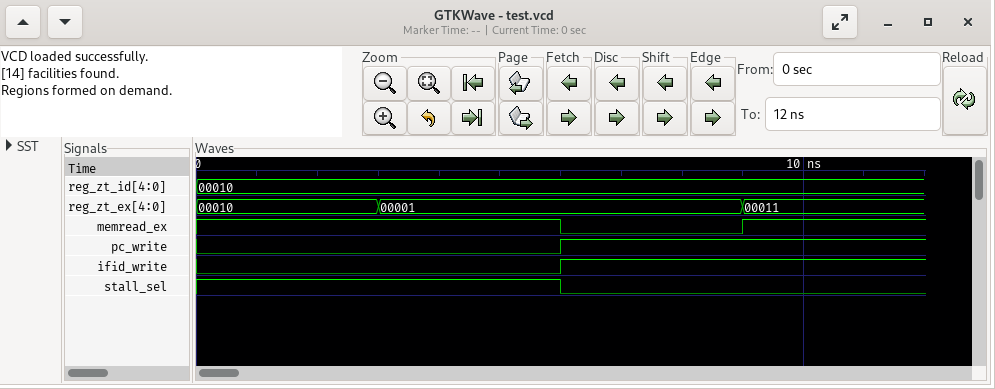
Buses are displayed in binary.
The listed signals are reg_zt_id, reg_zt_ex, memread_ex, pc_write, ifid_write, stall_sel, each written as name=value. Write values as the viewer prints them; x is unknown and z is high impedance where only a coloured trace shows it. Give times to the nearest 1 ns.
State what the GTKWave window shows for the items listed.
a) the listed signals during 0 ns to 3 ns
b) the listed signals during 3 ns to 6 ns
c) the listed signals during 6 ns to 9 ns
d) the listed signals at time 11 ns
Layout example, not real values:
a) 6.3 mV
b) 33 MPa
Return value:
a) reg_zt_id=00010, reg_zt_ex=00010, memread_ex=1, pc_write=0, ifid_write=0, stall_sel=1
b) reg_zt_id=00010, reg_zt_ex=00001, memread_ex=1, pc_write=0, ifid_write=0, stall_sel=1
c) reg_zt_id=00010, reg_zt_ex=00001, memread_ex=0, pc_write=1, ifid_write=1, stall_sel=0
d) reg_zt_id=00010, reg_zt_ex=00011, memread_ex=1, pc_write=1, ifid_write=1, stall_sel=0
